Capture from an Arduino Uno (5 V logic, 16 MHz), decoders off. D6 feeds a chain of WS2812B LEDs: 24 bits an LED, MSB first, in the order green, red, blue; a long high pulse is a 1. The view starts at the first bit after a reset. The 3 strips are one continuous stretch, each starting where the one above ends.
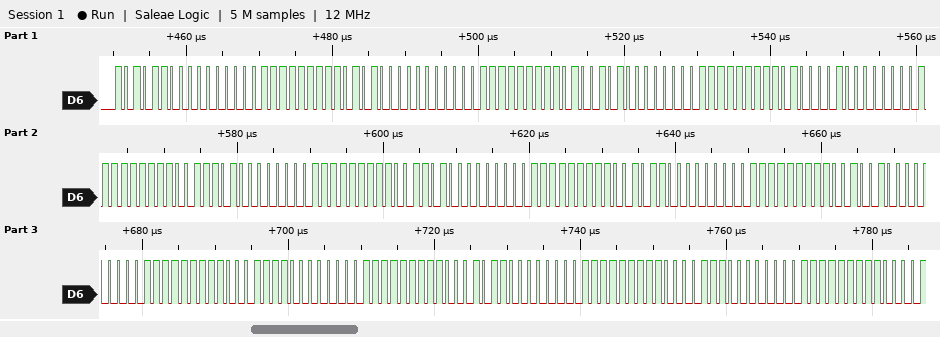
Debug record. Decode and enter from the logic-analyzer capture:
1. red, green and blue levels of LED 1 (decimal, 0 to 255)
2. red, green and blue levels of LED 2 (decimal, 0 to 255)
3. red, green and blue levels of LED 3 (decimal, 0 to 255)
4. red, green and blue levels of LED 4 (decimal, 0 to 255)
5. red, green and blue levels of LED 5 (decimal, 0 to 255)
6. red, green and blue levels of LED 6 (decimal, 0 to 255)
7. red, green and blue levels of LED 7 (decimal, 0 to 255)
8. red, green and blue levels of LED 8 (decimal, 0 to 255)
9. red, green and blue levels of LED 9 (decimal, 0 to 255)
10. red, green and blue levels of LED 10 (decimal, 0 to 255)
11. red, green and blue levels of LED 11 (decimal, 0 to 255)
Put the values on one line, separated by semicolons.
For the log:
0, 172, 255; 0, 168, 255; 0, 165, 255; 0, 161, 255; 0, 157, 255; 0, 154, 255; 0, 150, 255; 0, 146, 255; 0, 143, 255; 0, 139, 255; 0, 135, 255
